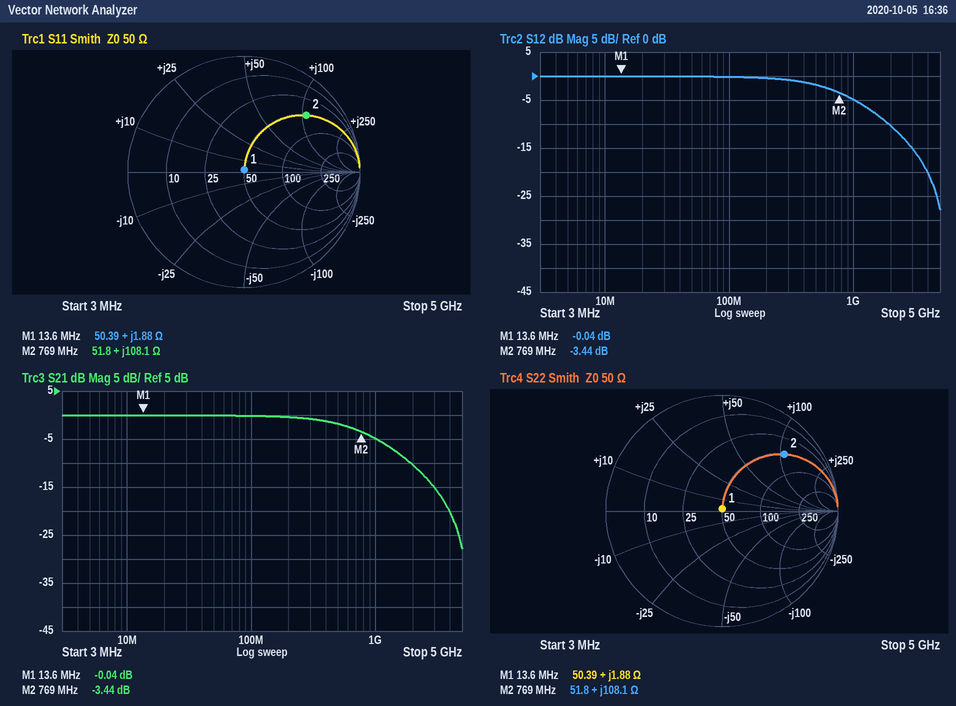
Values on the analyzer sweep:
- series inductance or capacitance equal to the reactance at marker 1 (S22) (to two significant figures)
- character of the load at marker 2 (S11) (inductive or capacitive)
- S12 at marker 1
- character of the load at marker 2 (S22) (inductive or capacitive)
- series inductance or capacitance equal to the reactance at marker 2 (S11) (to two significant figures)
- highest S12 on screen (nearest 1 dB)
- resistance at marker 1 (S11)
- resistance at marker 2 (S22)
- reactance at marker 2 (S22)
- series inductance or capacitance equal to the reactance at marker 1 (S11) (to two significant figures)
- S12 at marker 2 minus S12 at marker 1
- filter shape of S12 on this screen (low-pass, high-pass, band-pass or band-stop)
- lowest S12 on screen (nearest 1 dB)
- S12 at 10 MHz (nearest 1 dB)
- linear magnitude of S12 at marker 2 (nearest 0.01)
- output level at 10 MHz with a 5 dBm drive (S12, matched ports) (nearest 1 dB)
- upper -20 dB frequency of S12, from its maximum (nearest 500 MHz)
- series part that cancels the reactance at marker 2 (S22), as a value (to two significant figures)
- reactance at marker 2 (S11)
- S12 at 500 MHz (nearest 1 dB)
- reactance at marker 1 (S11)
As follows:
22 nH
inductive
-0.04 dB
inductive
22 nH
0 dB
50.39 Ω
51.8 Ω
+108.1 Ω
22 nH
-3.40 dB
low-pass
-28 dB
0 dB
0.67
5 dBm
4.0 GHz
1.9 pF
+108.1 Ω
-2 dB
+1.88 Ω
